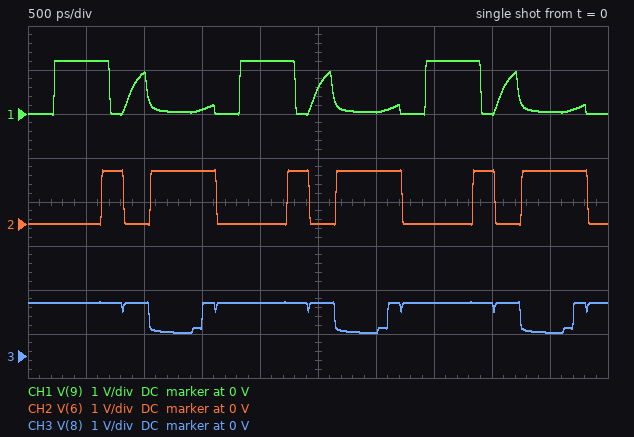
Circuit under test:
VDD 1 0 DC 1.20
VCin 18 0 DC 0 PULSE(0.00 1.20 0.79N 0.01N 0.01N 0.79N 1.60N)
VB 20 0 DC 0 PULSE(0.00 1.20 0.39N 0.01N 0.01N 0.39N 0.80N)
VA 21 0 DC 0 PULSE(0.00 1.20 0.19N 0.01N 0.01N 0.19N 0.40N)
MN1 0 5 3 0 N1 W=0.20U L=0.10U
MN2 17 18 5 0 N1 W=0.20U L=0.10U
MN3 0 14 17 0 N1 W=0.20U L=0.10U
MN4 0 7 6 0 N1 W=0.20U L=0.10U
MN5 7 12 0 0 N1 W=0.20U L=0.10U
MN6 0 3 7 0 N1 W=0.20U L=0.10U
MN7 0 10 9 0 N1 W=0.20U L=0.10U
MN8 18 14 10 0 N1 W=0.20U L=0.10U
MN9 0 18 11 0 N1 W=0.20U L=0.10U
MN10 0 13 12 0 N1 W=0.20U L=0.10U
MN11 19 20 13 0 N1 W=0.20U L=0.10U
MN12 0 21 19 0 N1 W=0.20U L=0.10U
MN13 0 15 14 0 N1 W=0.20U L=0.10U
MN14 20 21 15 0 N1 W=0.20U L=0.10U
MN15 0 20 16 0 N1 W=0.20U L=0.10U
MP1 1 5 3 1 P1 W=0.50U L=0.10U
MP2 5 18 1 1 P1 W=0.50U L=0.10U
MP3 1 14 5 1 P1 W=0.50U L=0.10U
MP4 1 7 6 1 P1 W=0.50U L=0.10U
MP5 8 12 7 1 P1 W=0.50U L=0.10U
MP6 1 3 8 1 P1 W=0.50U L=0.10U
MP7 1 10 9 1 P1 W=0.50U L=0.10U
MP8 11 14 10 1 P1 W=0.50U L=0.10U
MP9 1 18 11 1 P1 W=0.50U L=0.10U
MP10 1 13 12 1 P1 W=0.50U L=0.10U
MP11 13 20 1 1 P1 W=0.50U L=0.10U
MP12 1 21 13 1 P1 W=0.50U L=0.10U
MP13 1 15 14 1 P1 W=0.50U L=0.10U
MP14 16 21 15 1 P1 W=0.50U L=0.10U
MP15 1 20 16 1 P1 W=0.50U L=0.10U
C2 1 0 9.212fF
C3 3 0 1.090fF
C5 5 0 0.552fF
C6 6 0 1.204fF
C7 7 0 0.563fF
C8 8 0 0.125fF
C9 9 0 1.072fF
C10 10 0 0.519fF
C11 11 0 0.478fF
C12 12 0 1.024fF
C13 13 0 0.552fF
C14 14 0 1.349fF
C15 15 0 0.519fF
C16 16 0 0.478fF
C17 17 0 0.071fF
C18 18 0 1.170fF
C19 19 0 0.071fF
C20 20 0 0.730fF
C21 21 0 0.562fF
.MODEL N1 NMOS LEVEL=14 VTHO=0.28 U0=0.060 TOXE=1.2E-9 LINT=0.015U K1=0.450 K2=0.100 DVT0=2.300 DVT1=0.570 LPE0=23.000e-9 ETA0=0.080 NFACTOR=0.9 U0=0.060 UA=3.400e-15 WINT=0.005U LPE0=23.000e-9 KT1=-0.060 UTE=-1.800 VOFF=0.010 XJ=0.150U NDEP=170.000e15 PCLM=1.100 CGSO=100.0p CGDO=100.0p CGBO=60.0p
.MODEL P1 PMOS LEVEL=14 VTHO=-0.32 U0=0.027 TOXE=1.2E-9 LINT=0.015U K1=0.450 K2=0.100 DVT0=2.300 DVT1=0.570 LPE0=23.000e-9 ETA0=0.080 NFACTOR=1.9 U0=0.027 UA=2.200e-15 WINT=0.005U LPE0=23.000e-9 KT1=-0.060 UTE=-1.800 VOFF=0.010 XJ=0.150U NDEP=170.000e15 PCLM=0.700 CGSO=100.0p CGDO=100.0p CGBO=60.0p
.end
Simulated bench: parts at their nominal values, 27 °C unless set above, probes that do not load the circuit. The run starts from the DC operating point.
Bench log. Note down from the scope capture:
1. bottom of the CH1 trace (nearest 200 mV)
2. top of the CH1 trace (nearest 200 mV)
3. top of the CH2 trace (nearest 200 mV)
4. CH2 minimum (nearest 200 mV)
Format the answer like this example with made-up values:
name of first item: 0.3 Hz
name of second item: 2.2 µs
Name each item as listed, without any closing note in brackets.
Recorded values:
bottom of the CH1 trace: 0 V
top of the CH1 trace: 1.2 V
top of the CH2 trace: 1.2 V
CH2 minimum: 0 V
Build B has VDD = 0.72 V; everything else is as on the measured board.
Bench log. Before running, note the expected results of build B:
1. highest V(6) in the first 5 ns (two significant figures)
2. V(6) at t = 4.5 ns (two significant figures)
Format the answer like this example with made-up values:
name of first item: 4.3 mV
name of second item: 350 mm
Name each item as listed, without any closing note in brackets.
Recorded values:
highest V(6) in the first 5 ns: 780 mV
V(6) at t = 4.5 ns: 720 mV
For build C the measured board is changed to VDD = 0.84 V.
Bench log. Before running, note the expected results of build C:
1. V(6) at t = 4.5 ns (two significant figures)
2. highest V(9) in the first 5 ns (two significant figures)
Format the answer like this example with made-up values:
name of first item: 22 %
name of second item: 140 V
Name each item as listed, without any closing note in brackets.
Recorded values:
V(6) at t = 4.5 ns: 840 mV
highest V(9) in the first 5 ns: 890 mV
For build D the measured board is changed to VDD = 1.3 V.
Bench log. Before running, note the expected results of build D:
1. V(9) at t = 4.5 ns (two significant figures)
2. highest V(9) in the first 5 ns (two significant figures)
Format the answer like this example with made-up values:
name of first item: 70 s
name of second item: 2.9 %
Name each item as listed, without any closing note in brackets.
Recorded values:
V(9) at t = 4.5 ns: 71 mV
highest V(9) in the first 5 ns: 1.3 V
